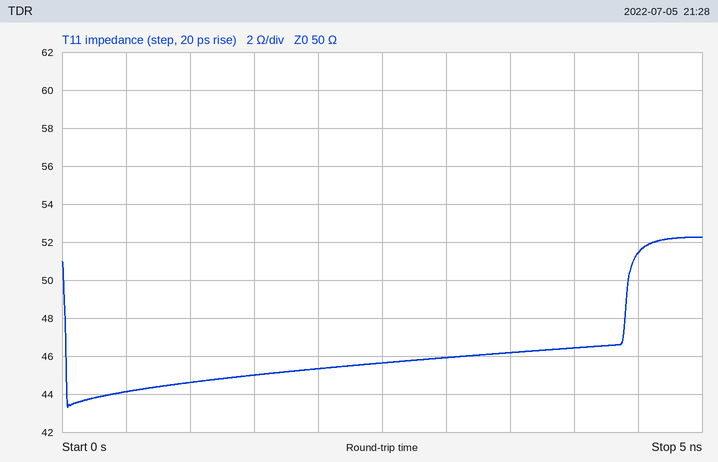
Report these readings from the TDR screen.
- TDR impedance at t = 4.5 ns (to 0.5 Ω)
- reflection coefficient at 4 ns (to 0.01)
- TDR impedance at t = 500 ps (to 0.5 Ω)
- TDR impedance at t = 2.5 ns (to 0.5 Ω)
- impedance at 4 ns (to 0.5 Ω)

51.5 Ω
-0.04
44.0 Ω
45.5 Ω
46.5 Ω
